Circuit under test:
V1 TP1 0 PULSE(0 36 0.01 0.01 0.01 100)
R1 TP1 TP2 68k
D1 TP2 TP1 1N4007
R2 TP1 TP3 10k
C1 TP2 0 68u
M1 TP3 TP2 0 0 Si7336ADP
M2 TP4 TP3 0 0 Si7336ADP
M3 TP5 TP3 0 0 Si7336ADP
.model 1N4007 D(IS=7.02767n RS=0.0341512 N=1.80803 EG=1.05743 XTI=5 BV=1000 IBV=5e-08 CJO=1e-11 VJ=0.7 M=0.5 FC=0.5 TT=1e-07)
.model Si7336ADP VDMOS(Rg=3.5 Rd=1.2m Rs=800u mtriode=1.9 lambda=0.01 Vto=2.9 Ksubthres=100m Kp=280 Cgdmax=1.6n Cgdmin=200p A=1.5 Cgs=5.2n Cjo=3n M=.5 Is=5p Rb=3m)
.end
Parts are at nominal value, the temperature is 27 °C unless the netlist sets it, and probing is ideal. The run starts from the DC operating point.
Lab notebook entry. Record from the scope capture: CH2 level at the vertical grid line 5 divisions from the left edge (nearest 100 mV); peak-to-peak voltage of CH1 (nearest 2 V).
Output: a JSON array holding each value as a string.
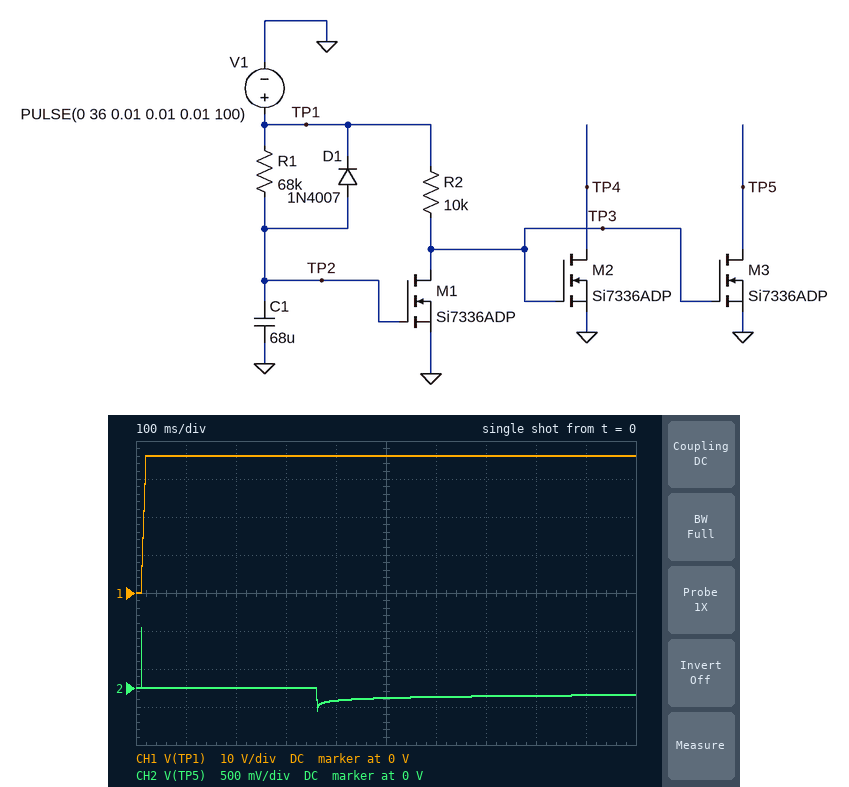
["-100 mV", "36 V"]
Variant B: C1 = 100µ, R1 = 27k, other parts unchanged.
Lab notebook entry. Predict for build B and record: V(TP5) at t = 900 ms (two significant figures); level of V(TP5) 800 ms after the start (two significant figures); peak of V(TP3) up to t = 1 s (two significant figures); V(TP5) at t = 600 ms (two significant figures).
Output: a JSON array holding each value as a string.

["-91 mV", "-95 mV", "36 V", "-110 mV"]
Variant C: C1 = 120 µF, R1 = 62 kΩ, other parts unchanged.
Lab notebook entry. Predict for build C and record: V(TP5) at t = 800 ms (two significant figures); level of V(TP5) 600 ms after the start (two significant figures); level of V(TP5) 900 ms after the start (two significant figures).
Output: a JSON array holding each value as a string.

["-120 mV", "-180 mV", "-110 mV"]
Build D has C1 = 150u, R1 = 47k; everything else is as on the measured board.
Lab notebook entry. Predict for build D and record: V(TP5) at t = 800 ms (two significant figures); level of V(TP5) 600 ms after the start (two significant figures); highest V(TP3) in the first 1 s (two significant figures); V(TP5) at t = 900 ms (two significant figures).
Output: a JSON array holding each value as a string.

["-120 mV", "-160 mV", "36 V", "-110 mV"]
